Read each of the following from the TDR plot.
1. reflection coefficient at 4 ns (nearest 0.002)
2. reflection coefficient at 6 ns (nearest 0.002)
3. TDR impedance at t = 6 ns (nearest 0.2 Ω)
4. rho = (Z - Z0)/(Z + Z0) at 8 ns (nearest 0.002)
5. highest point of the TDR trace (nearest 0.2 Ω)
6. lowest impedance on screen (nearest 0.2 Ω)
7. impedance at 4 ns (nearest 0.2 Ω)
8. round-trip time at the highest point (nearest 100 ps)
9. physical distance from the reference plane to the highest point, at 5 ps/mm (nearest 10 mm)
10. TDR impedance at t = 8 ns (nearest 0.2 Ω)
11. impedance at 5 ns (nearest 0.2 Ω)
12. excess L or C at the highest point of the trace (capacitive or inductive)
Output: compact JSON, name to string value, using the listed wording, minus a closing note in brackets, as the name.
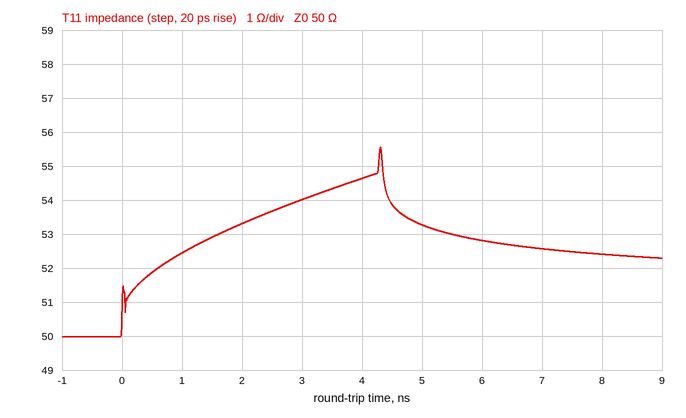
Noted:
{"reflection coefficient at 4 ns": "+0.044", "reflection coefficient at 6 ns": "+0.028", "TDR impedance at t = 6 ns": "52.8 Ω", "rho = (Z - Z0)/(Z + Z0) at 8 ns": "+0.024", "highest point of the TDR trace": "55.6 Ω", "lowest impedance on screen": "50.0 Ω", "impedance at 4 ns": "54.6 Ω", "round-trip time at the highest point": "4.3 ns", "physical distance from the reference plane to the highest point, at 5 ps/mm": "430 mm", "TDR impedance at t = 8 ns": "52.4 Ω", "impedance at 5 ns": "53.2 Ω", "excess L or C at the highest point of the trace": "inductive"}
